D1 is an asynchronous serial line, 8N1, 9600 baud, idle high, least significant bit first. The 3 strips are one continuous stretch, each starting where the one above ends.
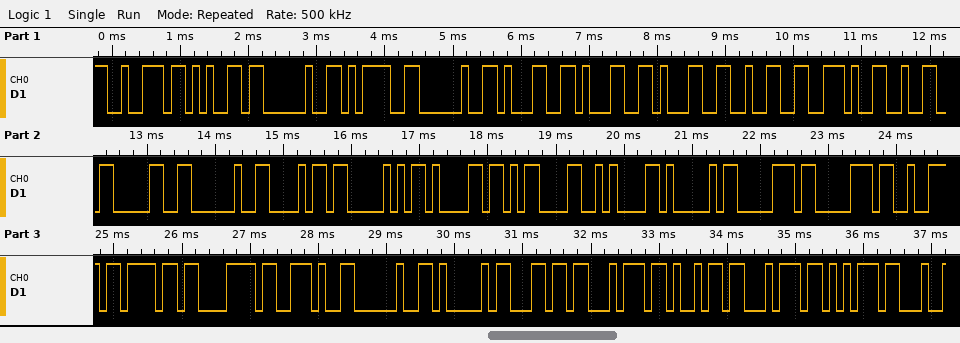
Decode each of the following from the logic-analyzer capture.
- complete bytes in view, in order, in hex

72 65 20 3D 20 31 31 31 32 2E 32 30 20 68 50 61 0D 0A 41 70 70 72 6F 78 2E 20 41 6C 74 69 74 75
